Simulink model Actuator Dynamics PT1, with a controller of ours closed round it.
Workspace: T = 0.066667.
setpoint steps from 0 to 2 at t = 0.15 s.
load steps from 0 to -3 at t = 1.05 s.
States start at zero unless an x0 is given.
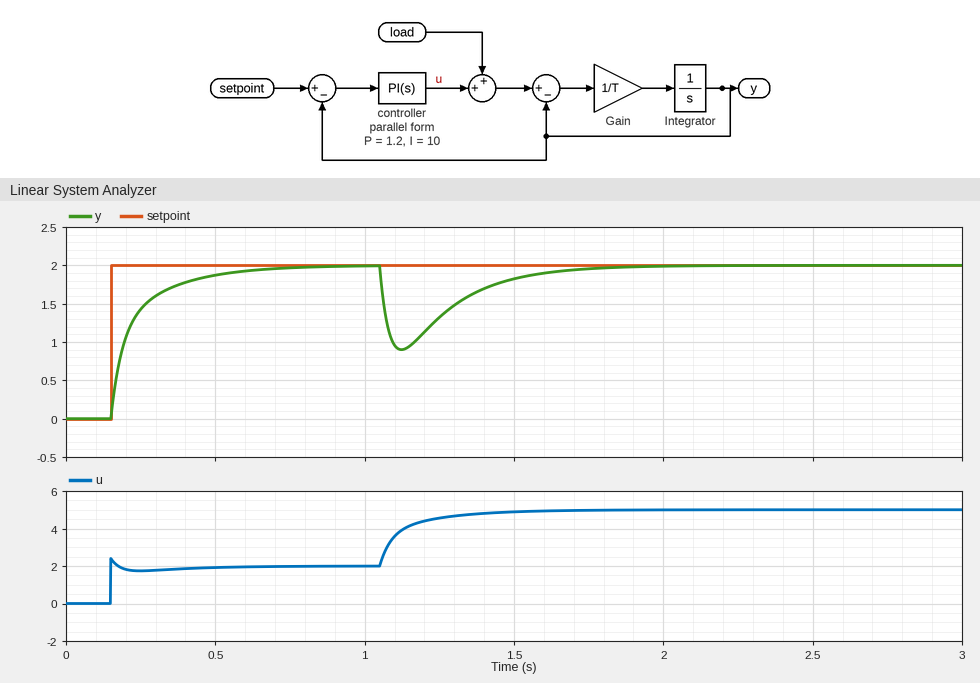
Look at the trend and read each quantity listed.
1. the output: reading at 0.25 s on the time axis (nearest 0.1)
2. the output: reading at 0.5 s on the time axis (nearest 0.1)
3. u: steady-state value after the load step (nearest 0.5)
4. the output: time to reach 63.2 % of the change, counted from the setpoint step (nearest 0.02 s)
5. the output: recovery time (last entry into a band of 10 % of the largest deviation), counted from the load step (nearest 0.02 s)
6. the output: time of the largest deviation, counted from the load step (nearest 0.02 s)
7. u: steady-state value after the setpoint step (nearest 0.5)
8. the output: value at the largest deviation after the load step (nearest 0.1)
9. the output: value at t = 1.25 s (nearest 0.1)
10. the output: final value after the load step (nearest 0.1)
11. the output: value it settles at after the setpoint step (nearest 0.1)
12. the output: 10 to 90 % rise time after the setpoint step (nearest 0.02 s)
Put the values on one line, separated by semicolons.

1.4; 1.9; 5.0; 0.08 s; 0.54 s; 0.08 s; 2.0; 0.9; 1.3; 2.0; 2.0; 0.26 s
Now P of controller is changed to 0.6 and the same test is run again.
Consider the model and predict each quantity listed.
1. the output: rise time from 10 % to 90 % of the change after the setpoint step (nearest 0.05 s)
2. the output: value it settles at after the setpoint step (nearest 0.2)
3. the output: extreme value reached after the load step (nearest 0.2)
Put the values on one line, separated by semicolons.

0.20 s; 2.0; 0.6
